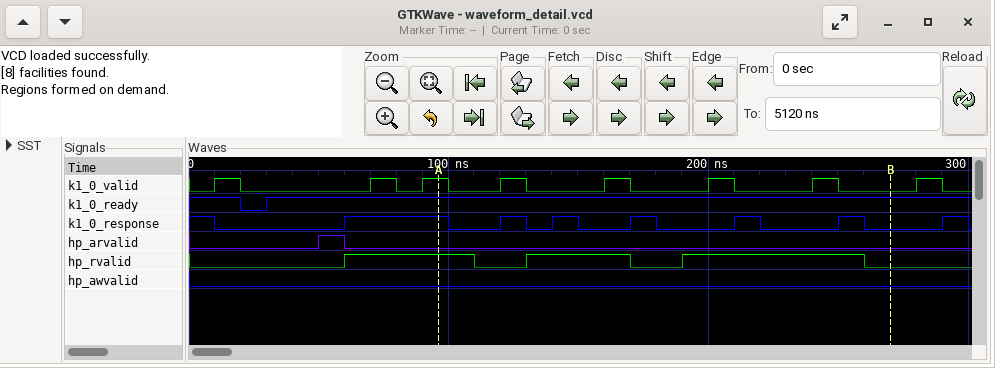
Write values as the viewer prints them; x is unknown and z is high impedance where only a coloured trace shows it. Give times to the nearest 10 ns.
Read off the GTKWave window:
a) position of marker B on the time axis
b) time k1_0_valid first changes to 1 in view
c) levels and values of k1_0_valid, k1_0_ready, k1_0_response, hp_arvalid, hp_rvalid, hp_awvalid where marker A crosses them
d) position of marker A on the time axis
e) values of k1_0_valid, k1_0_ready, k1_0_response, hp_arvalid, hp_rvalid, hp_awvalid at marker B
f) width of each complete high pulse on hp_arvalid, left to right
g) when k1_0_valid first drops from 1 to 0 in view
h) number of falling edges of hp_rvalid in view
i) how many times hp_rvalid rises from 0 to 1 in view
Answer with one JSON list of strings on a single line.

["270 ns", "10 ns", "k1_0_valid=1, k1_0_ready=1, k1_0_response=1, hp_arvalid=0, hp_rvalid=1, hp_awvalid=0", "100 ns", "k1_0_valid=0, k1_0_ready=1, k1_0_response=0, hp_arvalid=0, hp_rvalid=0, hp_awvalid=0", "10 ns", "20 ns", "3", "3"]
